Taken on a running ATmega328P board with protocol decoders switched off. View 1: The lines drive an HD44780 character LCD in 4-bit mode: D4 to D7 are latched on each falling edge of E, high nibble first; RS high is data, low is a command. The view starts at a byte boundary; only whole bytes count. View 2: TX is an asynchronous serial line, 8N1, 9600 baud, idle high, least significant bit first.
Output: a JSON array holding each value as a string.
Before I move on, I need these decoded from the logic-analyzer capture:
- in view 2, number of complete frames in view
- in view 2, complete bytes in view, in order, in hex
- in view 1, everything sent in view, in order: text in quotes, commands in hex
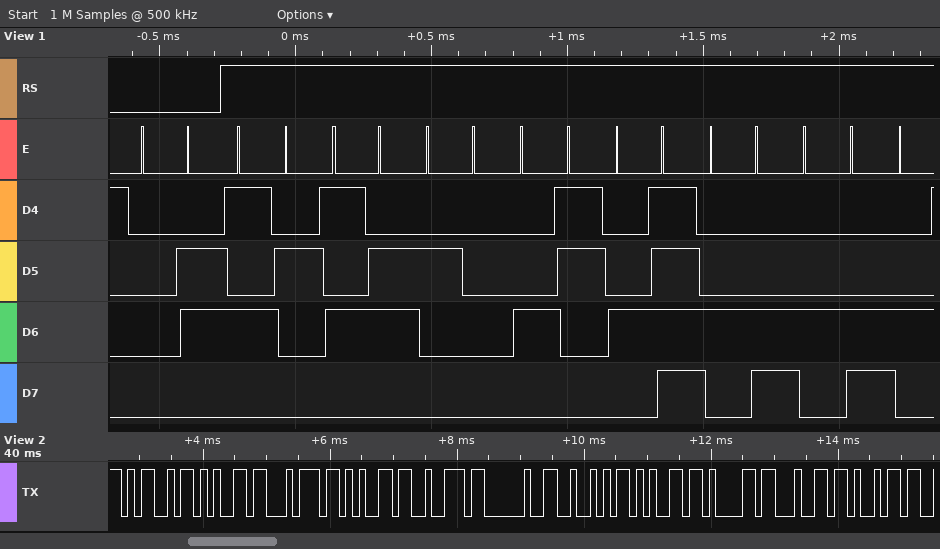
["11", "4D 65 74 65 72 20 52 65 61 64 69", "0x06 \"RV COLL\""]
